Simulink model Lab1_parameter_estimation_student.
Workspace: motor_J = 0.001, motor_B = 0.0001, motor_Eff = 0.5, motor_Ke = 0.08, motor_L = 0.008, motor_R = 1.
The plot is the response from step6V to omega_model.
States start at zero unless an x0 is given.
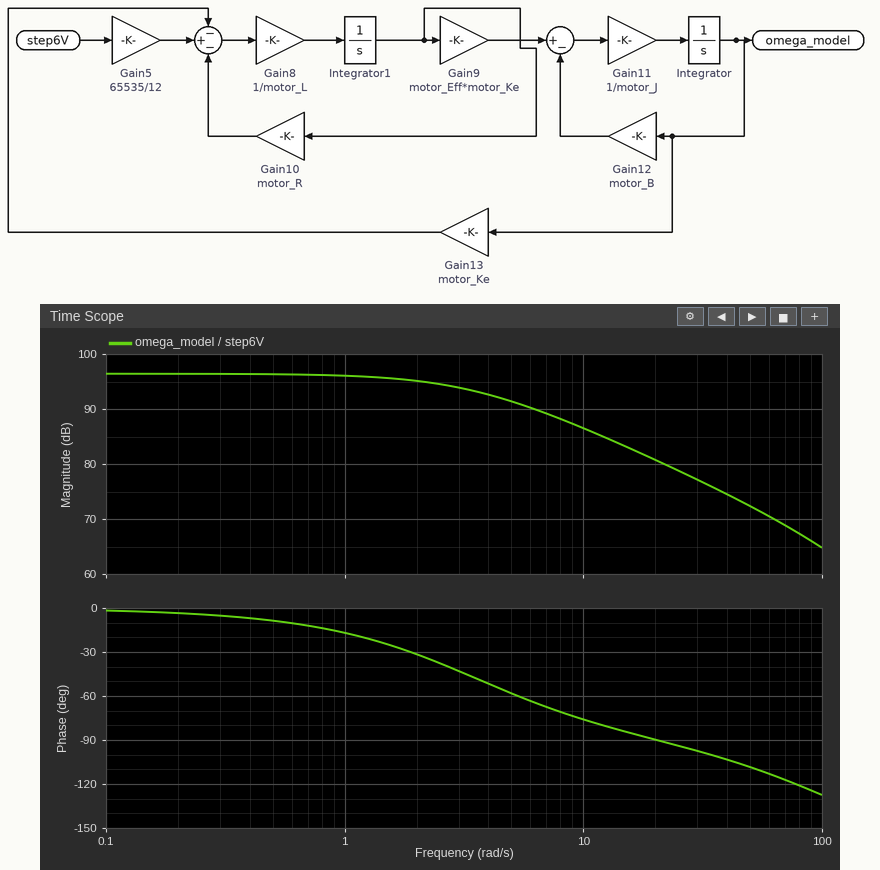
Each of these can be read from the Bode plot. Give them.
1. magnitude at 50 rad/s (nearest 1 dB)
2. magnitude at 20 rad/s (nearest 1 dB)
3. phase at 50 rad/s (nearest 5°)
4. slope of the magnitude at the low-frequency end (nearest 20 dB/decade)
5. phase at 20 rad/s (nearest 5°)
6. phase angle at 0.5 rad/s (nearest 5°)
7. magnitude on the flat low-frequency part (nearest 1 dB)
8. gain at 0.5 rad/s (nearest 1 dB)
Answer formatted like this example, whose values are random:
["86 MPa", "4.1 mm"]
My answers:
["72 dB", "81 dB", "-110°", "0 dB/decade", "-90°", "-10°", "96 dB", "96 dB"]
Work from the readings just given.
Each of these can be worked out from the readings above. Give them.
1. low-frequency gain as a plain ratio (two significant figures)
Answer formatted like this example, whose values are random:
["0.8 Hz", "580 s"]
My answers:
["63000"]
